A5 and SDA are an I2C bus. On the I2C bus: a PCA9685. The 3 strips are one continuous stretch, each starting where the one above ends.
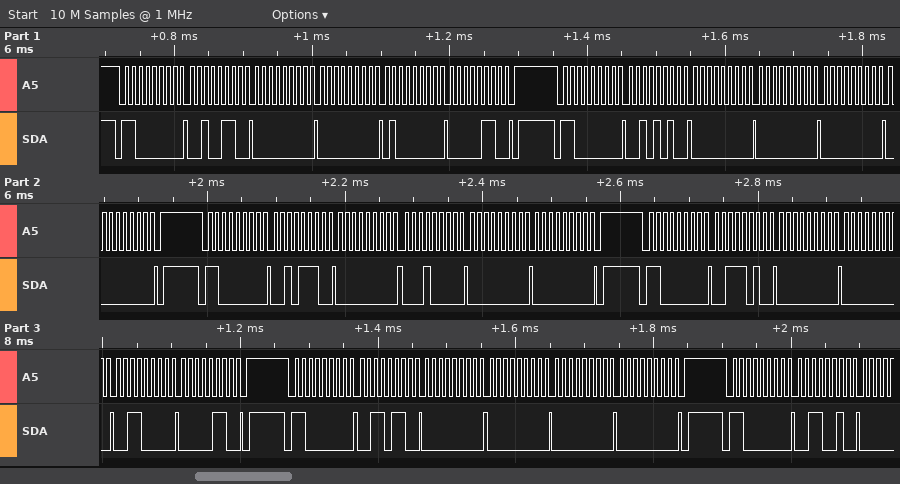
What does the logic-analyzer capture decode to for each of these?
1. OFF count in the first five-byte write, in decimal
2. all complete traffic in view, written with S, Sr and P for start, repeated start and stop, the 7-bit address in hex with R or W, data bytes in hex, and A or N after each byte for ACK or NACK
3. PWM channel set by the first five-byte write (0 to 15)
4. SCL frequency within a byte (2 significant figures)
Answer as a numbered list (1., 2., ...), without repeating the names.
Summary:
1. 1600
2. S 60W A 26 A 00 A 00 A 40 A 06 A P S 60W A 2A A 00 A 00 A 00 A 00 A P S 60W A 2E A 00 A 10 A 00 A 00 A P S 60W A 3A A 00 A 00 A 30 A 06 A P S 60W A 36 A 00 A 00 A 00 A 00 A P S 60W A 32 A
3. 8
4. 100 kHz
